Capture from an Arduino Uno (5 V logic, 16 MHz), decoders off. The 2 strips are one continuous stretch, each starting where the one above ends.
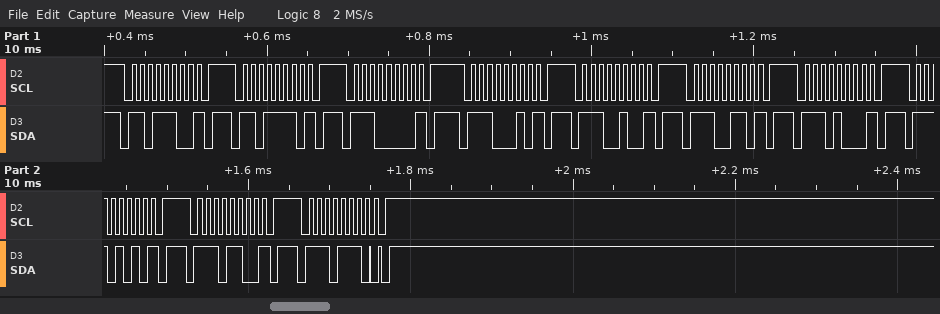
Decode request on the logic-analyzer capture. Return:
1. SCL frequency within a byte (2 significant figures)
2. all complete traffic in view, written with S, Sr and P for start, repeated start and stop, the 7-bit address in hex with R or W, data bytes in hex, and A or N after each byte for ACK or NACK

100 kHz
S 6EW N P S 6FW N P S 70W N P S 71W N P S 72W N P S 73W N P S 74W N P S 75W N P S 76W N P S 77W A P
